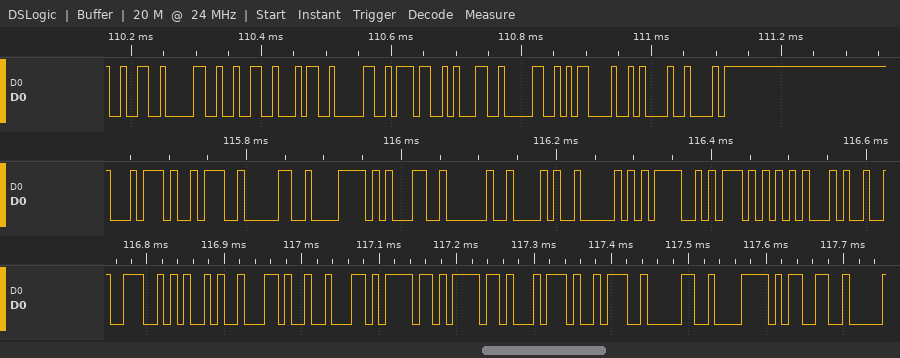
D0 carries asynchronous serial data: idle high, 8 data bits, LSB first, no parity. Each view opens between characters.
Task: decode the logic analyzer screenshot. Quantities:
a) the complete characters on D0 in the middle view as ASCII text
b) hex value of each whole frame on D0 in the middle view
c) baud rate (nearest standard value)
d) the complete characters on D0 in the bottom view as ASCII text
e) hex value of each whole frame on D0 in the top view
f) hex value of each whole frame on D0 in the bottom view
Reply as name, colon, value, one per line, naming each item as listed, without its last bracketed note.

the complete characters on D0 in the middle view as ASCII text: "t:0x1 (POWE"
hex value of each whole frame on D0 in the middle view: 74, 3A, 30, 78, 31, 20, 28, 50, 4F, 57, 45
baud rate: 115200 baud
the complete characters on D0 in the bottom view as ASCII text: "N),boot:0x3"
hex value of each whole frame on D0 in the top view: 32, 30, 32, 34, 30, 37, 31, 30, 0D, 0A, 42
hex value of each whole frame on D0 in the bottom view: 4E, 29, 2C, 62, 6F, 6F, 74, 3A, 30, 78, 33
